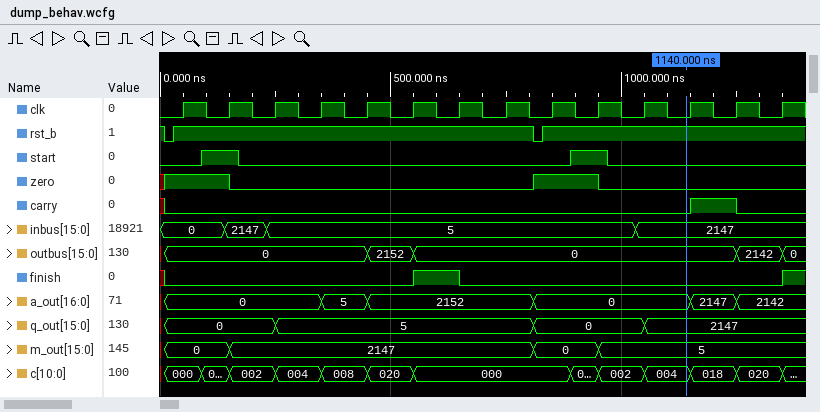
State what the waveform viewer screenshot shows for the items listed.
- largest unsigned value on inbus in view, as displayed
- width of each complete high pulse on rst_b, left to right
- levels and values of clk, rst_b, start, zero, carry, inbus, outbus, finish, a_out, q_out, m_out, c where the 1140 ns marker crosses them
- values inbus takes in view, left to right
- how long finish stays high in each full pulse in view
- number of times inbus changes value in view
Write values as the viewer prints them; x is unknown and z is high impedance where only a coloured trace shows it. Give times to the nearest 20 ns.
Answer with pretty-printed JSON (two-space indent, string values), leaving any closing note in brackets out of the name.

{
  "largest unsigned value on inbus in view, as displayed": "2147",
  "width of each complete high pulse on rst_b, left to right": "780 ns",
  "levels and values of clk, rst_b, start, zero, carry, inbus, outbus, finish, a_out, q_out, m_out, c where the 1140 ns marker crosses them": "clk=0, rst_b=1, start=0, zero=0, carry=0, inbus=2147, outbus=0, finish=0, a_out=0, q_out=2147, m_out=5, c=004",
  "values inbus takes in view, left to right": "0, 2147, 5, 2147",
  "how long finish stays high in each full pulse in view": "100 ns",
  "number of times inbus changes value in view": "3"
}
